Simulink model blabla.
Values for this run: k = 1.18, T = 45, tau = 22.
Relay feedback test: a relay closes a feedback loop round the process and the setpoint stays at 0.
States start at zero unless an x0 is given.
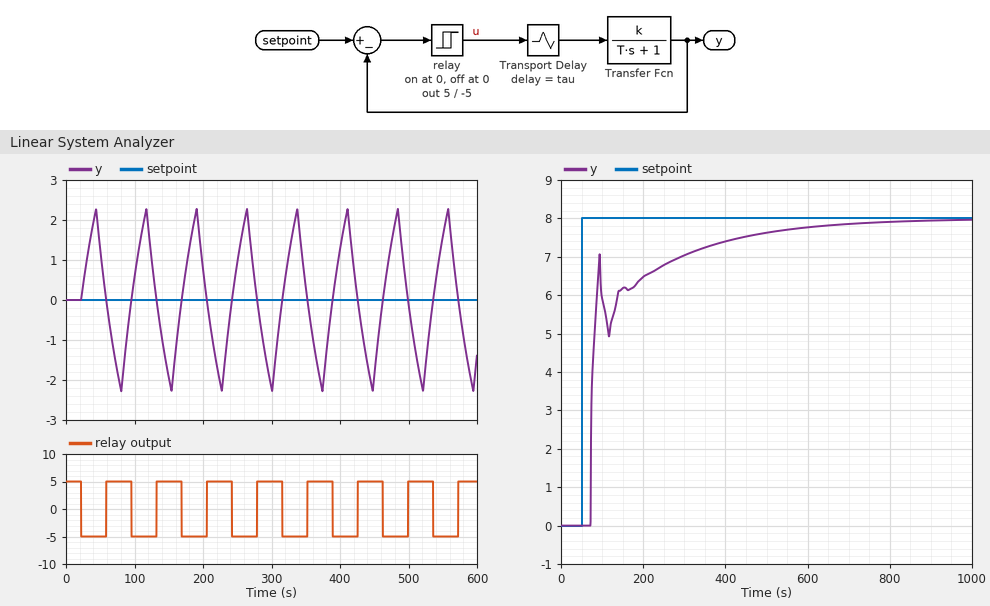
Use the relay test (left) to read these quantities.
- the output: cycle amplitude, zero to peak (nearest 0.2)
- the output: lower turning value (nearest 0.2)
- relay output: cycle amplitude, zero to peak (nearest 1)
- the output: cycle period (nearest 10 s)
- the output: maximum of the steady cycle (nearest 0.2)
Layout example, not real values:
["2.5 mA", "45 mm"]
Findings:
["2.2", "-2.2", "5", "70 s", "2.2"]
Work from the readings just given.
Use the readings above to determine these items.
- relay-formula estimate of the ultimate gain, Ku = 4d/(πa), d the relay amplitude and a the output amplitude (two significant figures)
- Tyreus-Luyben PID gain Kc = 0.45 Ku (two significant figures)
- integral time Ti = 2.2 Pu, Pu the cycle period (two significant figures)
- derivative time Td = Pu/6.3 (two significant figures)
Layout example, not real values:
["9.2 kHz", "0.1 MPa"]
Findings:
["2.9", "1.3", "150 s", "11 s"]
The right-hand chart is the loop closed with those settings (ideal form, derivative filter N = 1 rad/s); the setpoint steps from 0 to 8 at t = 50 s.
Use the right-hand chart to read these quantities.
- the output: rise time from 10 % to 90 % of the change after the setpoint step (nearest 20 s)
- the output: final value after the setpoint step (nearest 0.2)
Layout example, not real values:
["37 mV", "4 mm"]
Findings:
["260 s", "8.0"]
